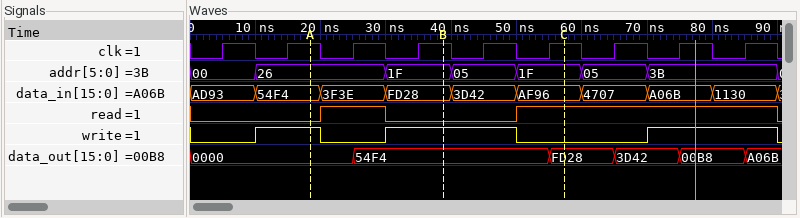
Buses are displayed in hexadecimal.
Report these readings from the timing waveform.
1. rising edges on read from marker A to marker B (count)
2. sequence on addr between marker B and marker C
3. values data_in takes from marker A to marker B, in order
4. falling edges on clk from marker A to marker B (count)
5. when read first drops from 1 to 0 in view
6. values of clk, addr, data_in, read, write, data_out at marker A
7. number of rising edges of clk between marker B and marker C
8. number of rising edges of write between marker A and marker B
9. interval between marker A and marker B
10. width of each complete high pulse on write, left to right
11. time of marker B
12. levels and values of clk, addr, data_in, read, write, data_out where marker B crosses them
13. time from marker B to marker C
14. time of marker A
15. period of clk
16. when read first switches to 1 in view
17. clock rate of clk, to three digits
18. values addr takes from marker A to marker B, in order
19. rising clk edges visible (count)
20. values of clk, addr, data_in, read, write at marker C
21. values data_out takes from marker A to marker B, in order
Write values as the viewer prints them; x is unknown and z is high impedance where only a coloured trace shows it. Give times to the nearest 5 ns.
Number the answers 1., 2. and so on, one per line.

1. 1
2. 1F, 05, 1F
3. 54F4, 3F3E, FD28
4. 2
5. 30 ns
6. clk=1, addr=26, data_in=54F4, read=0, write=1, data_out=0000
7. 2
8. 1
9. 20 ns
10. 10 ns, 20 ns, 20 ns
11. 40 ns
12. clk=1, addr=1F, data_in=FD28, read=0, write=1, data_out=54F4
13. 20 ns
14. 20 ns
15. 10 ns
16. 20 ns
17. 100 MHz
18. 26, 1F
19. 9
20. clk=1, addr=1F, data_in=AF96, read=1, write=0
21. 0000, 54F4
